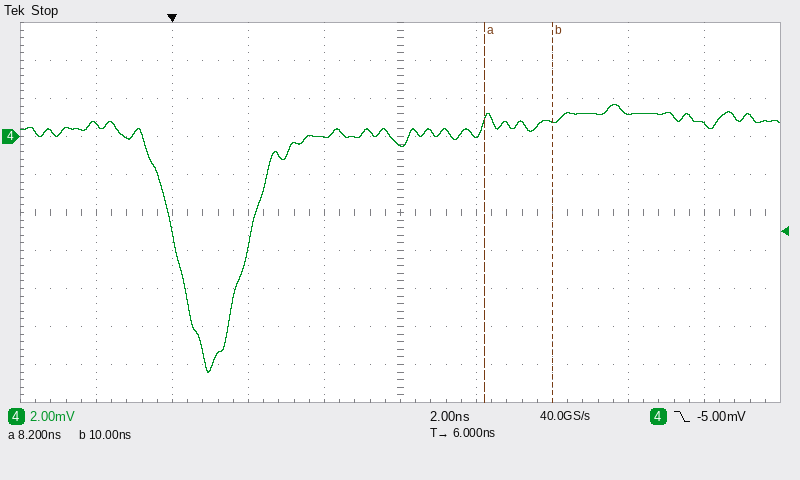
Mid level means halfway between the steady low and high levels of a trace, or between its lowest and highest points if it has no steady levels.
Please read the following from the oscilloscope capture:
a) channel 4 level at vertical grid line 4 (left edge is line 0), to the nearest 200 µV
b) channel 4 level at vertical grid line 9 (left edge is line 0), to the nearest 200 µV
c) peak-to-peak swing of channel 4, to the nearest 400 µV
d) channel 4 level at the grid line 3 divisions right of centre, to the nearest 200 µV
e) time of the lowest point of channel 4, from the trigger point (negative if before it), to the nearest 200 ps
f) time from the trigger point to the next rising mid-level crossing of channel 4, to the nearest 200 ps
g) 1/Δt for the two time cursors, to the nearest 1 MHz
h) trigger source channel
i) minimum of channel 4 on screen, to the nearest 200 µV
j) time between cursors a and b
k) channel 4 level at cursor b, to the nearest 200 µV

0.0 mV
600 µV
14.0 mV
1.2 mV
+1.0 ns
2.0 ns
556 MHz
channel 4
-12.4 mV
1.8 ns
800 µV
